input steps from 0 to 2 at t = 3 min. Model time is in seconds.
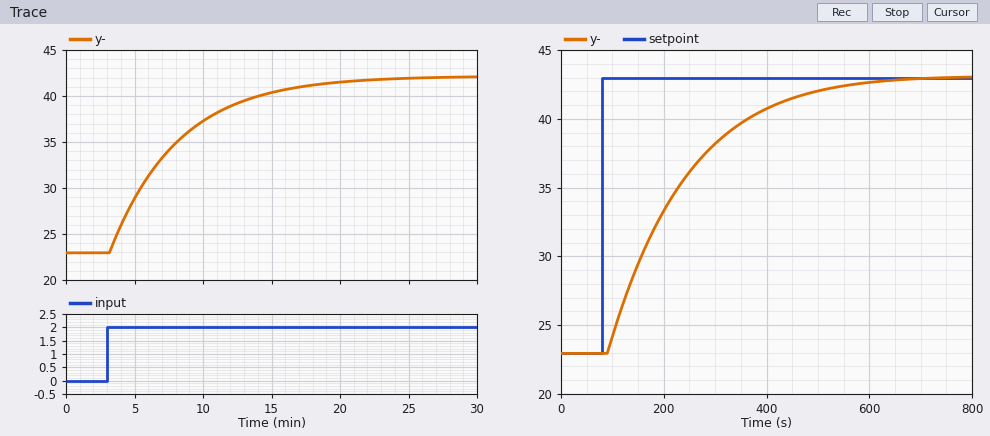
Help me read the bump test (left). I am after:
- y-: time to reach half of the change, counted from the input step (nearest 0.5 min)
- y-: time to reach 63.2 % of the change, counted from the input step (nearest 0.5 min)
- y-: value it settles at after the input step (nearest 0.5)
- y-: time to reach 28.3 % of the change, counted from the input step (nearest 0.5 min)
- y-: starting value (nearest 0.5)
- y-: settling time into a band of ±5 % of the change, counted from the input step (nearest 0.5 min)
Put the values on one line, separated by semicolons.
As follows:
3.5 min; 5.0 min; 42.0; 2.0 min; 23.0; 15.0 min
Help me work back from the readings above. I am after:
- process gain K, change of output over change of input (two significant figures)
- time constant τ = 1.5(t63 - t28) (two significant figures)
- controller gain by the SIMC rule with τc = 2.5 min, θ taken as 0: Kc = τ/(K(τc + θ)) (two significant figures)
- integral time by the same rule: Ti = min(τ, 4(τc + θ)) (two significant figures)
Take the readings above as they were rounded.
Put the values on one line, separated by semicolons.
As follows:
9.5; 4.5 min; 0.19; 4.5 min
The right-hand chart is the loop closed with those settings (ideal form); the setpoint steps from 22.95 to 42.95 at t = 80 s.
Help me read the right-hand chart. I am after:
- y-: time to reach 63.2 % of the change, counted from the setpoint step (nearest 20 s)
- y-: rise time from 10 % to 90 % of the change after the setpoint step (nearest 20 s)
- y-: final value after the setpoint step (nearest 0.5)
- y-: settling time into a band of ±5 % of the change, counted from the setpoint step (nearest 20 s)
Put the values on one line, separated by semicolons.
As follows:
160 s; 300 s; 43.0; 420 s
